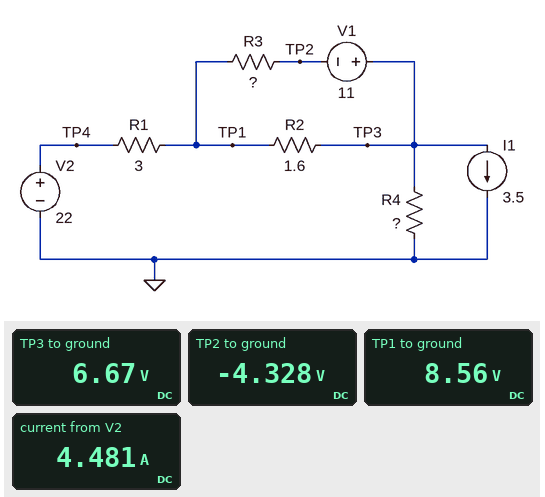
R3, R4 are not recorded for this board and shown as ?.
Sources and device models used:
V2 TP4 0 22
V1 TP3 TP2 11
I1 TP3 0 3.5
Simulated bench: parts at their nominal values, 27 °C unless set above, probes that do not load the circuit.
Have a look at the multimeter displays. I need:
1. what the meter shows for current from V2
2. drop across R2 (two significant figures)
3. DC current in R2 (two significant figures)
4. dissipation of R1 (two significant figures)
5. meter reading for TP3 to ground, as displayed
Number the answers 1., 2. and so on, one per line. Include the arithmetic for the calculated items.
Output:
1. 4.481 A
2. 8.56 V - 6.67 V = 1.9 V
3. (8.56 V - 6.67 V) / 1.6 Ω = 1.2 A
4. (22 V - 8.56 V)^2 / 3 Ω = 60 W
5. 6.67 V
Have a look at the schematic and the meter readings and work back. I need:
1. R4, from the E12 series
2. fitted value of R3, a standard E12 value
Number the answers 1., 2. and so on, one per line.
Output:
1. 6.8 Ω
2. 3.9 Ω
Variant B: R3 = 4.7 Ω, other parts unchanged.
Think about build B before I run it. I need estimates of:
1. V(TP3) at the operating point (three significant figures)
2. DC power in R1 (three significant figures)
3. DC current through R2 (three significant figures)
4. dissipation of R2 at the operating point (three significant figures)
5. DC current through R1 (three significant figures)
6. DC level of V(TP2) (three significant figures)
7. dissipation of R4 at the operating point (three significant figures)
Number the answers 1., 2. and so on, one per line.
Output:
1. 6.26 V
2. 58.6 W
3. 1.55 A
4. 3.85 W
5. 4.42 A
6. -4.74 V
7. 5.76 W
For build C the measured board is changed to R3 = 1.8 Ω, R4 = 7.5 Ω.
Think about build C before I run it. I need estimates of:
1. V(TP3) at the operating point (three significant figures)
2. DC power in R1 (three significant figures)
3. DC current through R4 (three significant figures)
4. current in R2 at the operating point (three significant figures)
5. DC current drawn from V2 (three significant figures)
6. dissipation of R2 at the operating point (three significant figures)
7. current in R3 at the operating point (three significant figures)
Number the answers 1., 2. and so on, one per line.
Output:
1. 9.06 V
2. 66.5 W
3. 1.21 A
4. 743 mA
5. 4.71 A
6. 882 mW
7. 5.45 A
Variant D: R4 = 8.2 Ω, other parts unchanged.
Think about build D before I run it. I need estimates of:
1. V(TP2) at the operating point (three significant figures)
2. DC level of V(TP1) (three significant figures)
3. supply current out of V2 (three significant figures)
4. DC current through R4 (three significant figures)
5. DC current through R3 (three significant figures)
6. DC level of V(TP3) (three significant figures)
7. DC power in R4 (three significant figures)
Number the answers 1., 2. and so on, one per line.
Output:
1. -3.87 V
2. 8.89 V
3. 4.37 A
4. 870 mA
5. 3.27 A
6. 7.13 V
7. 6.20 W
